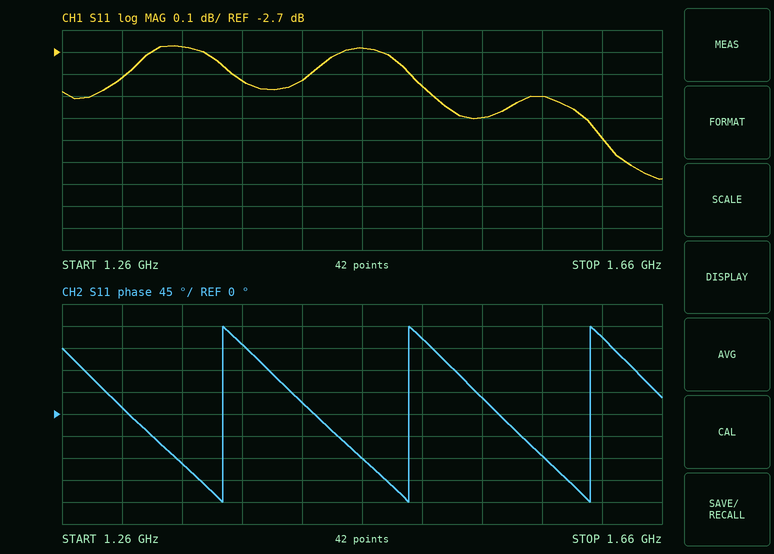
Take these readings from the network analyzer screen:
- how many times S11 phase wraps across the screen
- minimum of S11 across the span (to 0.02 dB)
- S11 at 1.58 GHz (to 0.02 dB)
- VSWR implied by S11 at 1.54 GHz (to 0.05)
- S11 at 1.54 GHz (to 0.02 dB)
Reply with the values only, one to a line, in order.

3
-3.28 dB
-2.90 dB
5.85
-3.00 dB
